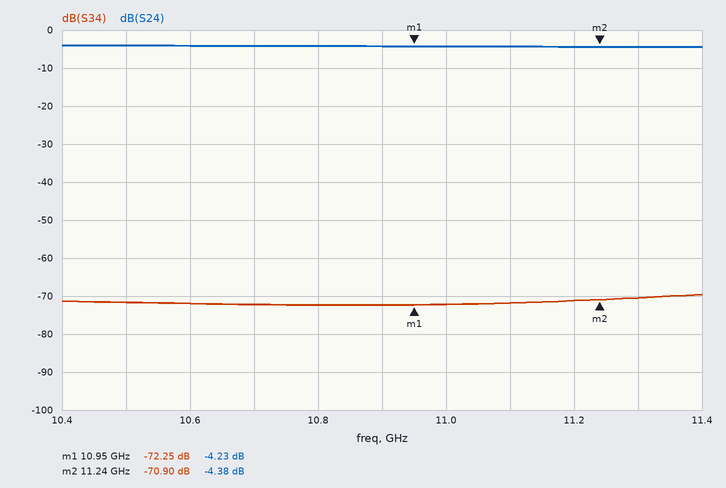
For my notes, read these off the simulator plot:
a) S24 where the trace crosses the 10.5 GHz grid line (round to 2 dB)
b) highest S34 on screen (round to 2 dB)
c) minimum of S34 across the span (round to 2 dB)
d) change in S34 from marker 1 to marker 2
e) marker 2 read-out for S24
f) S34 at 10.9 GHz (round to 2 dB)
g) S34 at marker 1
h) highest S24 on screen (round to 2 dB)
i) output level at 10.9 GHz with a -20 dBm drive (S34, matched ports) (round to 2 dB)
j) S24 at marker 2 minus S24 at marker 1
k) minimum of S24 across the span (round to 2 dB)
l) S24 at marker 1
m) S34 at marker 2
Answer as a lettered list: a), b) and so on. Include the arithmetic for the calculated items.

a) -4 dB
b) -70 dB
c) -72 dB
d) -70.9 − (-72.25) = 1.35 dB
e) -4.38 dB
f) -72 dB
g) -72.25 dB
h) -4 dB
i) -20 dBm + (-72 dB) = -92 dBm
j) -4.38 − (-4.23) = -0.15 dB
k) -4 dB
l) -4.23 dB
m) -70.90 dB
